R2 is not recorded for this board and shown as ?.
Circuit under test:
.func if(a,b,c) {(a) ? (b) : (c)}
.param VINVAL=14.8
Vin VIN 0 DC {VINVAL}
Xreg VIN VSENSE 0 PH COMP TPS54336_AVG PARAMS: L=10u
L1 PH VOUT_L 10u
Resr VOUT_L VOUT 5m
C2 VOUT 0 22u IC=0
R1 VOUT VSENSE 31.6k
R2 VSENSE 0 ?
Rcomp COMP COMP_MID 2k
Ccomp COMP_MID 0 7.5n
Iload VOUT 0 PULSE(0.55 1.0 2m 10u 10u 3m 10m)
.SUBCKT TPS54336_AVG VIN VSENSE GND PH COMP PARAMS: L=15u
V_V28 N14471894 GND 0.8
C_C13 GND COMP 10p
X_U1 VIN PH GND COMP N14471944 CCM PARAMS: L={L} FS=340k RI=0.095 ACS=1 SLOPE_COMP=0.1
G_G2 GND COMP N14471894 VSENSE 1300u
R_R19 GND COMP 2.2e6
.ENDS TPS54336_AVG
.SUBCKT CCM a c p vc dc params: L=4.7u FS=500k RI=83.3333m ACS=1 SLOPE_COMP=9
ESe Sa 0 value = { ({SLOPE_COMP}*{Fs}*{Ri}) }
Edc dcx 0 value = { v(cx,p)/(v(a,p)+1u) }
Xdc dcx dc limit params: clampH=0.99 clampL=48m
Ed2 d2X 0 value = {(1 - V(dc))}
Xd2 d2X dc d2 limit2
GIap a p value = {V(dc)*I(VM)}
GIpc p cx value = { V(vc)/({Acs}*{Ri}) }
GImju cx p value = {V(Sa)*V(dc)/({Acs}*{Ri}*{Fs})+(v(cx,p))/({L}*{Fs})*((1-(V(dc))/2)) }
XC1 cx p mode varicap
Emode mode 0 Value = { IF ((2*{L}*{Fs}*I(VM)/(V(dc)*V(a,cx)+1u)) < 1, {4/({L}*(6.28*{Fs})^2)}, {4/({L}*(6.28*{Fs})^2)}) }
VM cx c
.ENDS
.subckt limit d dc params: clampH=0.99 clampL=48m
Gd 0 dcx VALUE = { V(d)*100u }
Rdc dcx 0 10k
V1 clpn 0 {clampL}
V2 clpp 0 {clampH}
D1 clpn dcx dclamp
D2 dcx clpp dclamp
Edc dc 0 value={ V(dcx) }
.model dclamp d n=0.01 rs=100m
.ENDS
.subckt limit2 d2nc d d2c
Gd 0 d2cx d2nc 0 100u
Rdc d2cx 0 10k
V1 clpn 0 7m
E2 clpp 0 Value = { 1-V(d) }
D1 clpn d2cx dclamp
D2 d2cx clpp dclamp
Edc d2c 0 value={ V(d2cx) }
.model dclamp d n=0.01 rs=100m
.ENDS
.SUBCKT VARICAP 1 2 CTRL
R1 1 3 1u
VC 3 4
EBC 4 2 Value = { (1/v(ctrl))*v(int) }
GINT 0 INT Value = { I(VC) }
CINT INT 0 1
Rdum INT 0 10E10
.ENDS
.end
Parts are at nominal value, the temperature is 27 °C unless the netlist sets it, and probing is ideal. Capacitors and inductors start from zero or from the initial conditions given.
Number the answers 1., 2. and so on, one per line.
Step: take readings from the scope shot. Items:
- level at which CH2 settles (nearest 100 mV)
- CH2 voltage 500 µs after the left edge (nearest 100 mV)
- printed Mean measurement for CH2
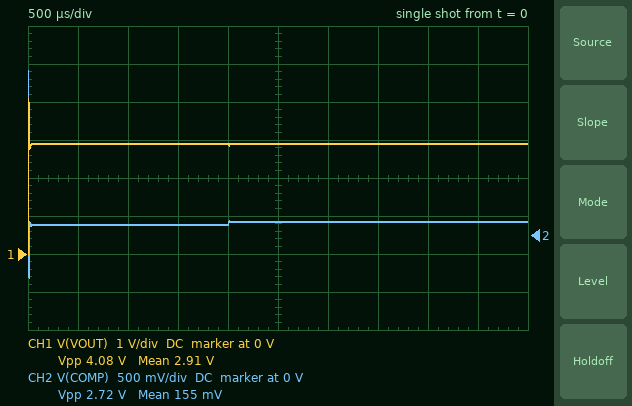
1. 200 mV
2. 100 mV
3. 155 mV
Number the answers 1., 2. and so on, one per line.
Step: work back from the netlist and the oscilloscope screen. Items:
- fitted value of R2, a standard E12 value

1. 12 kΩ
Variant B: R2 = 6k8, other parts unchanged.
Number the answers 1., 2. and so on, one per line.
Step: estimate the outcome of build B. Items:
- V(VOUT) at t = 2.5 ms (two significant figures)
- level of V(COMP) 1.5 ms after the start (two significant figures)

1. 4.5 V
2. 160 mV
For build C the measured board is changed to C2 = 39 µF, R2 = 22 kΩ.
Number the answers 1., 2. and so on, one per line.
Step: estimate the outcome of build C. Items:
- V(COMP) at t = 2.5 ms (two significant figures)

1. 150 mV
